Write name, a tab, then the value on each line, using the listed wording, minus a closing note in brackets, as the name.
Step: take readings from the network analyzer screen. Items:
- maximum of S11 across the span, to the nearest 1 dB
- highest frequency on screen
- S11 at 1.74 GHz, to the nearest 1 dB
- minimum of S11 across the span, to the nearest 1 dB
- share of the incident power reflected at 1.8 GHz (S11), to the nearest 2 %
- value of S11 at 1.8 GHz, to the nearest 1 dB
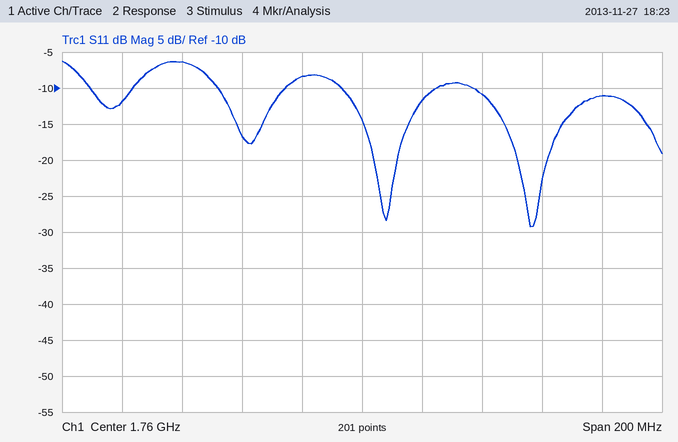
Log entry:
maximum of S11 across the span, to the nearest 1 dB	-6 dB
highest frequency on screen	1.86 GHz
S11 at 1.74 GHz, to the nearest 1 dB	-8 dB
minimum of S11 across the span, to the nearest 1 dB	-29 dB
share of the incident power reflected at 1.8 GHz (S11), to the nearest 2 %	8 %
value of S11 at 1.8 GHz, to the nearest 1 dB	-11 dB
